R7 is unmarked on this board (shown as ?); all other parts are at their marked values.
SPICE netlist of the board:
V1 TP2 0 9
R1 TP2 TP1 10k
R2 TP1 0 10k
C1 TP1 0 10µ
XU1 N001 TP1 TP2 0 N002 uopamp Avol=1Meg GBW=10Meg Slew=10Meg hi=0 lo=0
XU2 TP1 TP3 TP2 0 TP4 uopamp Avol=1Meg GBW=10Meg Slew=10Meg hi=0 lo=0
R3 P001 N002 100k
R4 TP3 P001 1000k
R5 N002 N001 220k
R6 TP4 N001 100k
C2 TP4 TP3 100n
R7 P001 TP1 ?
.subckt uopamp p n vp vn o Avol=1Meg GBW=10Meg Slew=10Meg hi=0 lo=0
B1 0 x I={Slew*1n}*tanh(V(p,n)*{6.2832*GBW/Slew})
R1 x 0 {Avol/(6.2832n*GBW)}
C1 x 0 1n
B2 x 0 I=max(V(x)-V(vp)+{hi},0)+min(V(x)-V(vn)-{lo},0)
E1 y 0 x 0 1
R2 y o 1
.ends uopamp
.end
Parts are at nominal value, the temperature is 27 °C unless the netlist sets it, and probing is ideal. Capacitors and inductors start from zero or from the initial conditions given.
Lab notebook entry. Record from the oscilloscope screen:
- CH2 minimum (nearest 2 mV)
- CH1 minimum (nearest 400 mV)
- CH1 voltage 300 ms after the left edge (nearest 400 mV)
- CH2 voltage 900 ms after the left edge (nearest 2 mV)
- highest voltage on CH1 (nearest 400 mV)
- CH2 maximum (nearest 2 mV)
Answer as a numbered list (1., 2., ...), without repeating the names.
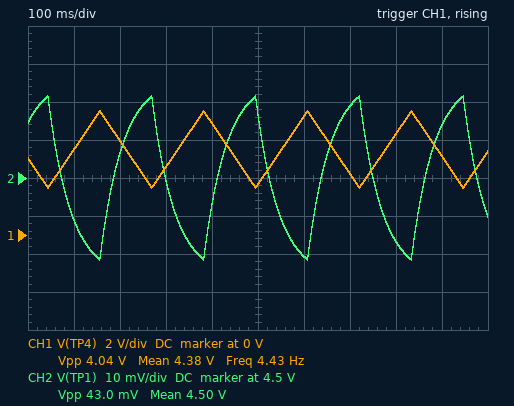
1. 4.478 V
2. 2.4 V
3. 3.6 V
4. 4.514 V
5. 6.4 V
6. 4.522 V
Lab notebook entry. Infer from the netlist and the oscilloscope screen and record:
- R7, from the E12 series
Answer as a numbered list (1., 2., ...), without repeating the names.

1. 680 kΩ
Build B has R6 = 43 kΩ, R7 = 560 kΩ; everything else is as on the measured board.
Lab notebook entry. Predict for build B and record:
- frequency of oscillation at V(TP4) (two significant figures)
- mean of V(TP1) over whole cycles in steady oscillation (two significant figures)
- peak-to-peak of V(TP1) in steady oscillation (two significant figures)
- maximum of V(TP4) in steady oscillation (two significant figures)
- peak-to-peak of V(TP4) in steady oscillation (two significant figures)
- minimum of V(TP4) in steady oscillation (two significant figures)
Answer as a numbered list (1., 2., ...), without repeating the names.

1. 10 Hz
2. 4.5 V
3. 29 mV
4. 5.4 V
5. 1.7 V
6. 3.6 V
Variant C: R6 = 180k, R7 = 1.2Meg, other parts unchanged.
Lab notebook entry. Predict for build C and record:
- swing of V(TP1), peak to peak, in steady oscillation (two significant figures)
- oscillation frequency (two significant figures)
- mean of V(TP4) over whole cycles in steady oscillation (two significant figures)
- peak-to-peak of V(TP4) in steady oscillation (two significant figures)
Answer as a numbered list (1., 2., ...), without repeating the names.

1. 30 mV
2. 2.6 Hz
3. 4.5 V
4. 7.3 V
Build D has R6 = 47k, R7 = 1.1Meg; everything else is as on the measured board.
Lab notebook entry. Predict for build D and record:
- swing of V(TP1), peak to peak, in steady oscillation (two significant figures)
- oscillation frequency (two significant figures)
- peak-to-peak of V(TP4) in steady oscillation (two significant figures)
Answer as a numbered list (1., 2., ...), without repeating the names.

1. 16 mV
2. 9.9 Hz
3. 1.9 V
